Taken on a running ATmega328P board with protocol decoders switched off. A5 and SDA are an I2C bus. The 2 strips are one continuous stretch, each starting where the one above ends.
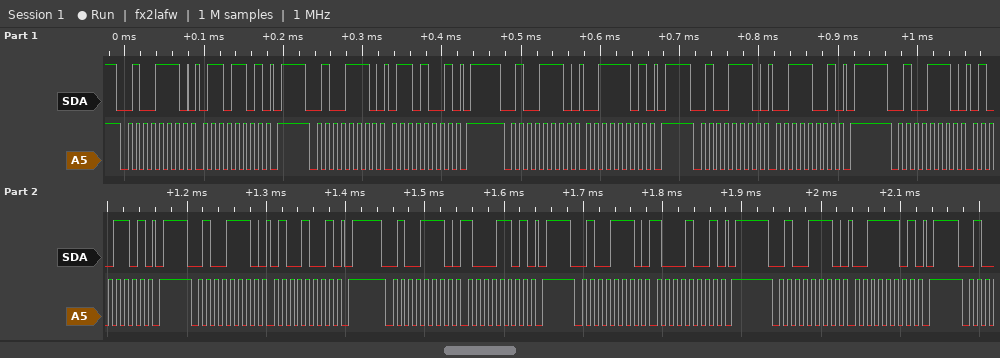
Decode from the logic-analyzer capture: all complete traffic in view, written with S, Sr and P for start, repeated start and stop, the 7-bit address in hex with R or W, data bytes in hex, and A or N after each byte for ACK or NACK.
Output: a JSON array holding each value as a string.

["S 27W A 6D A P S 27W A 69 A P S 27W A 3D A P S 27W A 39 A P S 27W A 4D A P S 27W A 49 A P S 27W A 8D A P S 27W A 89 A P S 27W A 3D A P"]
